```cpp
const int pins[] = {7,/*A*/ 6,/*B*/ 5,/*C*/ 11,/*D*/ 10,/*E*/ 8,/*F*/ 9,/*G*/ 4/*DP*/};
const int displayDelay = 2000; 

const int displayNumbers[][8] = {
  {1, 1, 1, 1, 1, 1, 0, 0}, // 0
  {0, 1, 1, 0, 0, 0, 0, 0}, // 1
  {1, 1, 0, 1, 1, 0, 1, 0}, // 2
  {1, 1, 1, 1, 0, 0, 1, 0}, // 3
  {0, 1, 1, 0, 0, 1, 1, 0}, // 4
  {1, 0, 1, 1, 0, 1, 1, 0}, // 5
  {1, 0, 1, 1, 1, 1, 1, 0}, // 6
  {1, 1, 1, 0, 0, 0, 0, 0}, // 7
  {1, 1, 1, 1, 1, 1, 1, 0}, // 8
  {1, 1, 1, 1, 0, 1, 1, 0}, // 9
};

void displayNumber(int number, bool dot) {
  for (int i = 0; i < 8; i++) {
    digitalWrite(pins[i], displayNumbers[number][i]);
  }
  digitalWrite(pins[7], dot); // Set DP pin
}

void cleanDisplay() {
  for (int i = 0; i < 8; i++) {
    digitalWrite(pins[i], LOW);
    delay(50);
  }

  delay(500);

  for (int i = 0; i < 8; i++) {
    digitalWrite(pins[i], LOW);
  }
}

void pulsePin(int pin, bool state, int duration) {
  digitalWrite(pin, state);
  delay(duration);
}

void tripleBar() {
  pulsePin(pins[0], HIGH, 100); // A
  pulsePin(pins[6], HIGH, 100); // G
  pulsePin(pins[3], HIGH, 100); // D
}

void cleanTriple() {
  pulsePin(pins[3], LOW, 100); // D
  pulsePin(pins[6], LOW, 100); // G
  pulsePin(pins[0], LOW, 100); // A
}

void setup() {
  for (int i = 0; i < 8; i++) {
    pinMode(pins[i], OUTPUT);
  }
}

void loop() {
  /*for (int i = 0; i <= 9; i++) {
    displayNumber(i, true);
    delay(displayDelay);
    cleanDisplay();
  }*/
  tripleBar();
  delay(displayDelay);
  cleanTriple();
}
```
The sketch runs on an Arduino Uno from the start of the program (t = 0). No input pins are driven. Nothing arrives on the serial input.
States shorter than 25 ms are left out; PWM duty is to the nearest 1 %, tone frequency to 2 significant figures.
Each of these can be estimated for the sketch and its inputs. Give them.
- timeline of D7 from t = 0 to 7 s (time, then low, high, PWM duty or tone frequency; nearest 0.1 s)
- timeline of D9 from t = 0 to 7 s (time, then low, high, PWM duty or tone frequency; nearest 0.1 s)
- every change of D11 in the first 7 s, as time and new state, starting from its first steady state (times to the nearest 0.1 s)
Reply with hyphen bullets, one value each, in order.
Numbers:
- 0 s high; 2.5 s low; 2.6 s high; 5.1 s low; 5.2 s high
- 0 s low; 0.1 s high; 2.4 s low; 2.7 s high; 5 s low; 5.3 s high
- 0 s low; 0.2 s high; 2.3 s low; 2.8 s high; 4.9 s low; 5.4 s high
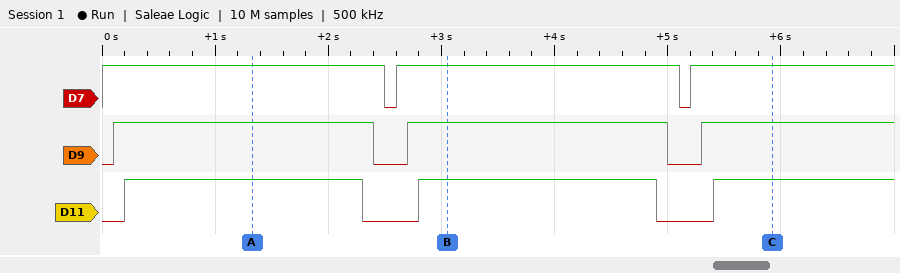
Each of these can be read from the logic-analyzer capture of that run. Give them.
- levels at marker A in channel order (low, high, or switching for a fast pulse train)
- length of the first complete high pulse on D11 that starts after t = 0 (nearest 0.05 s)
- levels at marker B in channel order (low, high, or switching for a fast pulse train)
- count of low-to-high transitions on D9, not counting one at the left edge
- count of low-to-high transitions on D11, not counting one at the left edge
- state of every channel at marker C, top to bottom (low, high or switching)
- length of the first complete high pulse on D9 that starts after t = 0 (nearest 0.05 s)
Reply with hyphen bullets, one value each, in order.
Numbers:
- D7 high, D9 high, D11 high
- 2.10 s
- D7 high, D9 high, D11 high
- 3
- 3
- D7 high, D9 high, D11 high
- 2.30 s
